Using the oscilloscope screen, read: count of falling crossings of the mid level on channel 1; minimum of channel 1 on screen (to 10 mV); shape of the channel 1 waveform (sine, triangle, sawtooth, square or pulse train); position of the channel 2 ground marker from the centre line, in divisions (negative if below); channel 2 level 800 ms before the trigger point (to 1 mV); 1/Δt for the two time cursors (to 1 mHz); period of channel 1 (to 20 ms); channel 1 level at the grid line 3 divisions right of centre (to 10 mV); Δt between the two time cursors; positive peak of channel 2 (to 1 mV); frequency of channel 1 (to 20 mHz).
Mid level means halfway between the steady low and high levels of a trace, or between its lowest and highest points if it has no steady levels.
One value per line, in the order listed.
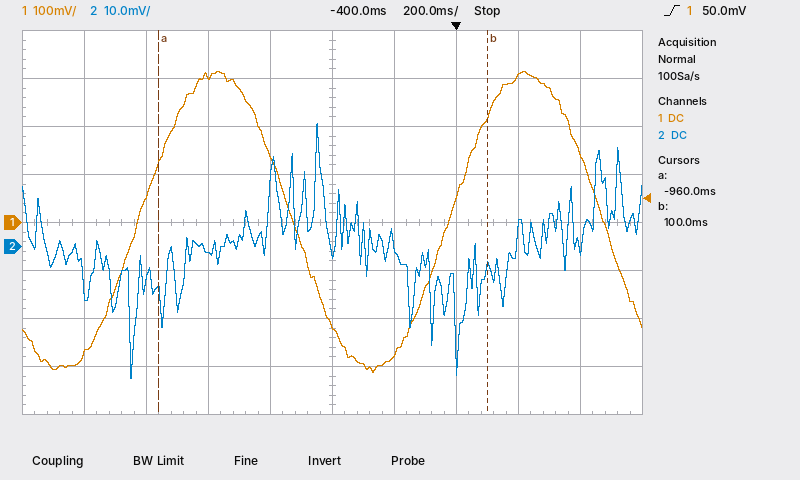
2
-310 mV
sine
-0.5 div
-1 mV
943 mHz
1.00 s
300 mV
1.06 s
26 mV
1.00 Hz
